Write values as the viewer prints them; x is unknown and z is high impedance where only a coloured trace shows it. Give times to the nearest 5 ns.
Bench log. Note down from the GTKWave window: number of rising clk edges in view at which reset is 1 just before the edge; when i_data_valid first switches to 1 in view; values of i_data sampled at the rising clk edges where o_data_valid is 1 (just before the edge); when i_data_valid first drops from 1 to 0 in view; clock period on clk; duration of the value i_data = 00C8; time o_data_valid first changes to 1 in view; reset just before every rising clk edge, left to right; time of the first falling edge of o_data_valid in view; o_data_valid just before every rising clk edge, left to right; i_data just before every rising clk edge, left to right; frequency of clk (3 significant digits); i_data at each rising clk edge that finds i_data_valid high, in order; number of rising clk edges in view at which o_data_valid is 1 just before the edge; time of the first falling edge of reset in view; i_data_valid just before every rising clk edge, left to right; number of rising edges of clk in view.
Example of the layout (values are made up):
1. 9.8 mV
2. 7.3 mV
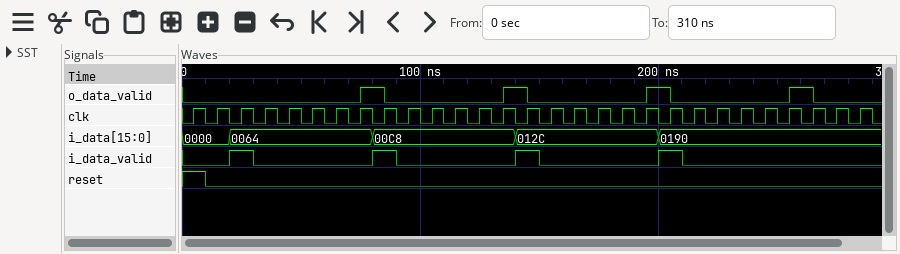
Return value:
1. 1
2. 20 ns
3. 00C8, 012C, 0190, 0190
4. 30 ns
5. 10 ns
6. 60 ns
7. 75 ns
8. 1 0 0 0 0 0 0 0 0 0 0 0 0 0 0 0 0 0 0 0 0 0 0 0 0 0 0 0 0
9. 85 ns
10. 0 0 0 0 0 0 0 0 1 0 0 0 0 0 1 0 0 0 0 0 1 0 0 0 0 0 1 0 0
11. 0000, 0000, 0064, 0064, 0064, 0064, 0064, 0064, 00C8, 00C8, 00C8, 00C8, 00C8, 00C8, 012C, 012C, 012C, 012C, 012C, 012C, 0190, 0190, 0190, 0190, 0190, 0190, 0190, 0190, 0190
12. 100 MHz
13. 0064, 00C8, 012C, 0190
14. 4
15. 10 ns
16. 0 0 1 0 0 0 0 0 1 0 0 0 0 0 1 0 0 0 0 0 1 0 0 0 0 0 0 0 0
17. 29
